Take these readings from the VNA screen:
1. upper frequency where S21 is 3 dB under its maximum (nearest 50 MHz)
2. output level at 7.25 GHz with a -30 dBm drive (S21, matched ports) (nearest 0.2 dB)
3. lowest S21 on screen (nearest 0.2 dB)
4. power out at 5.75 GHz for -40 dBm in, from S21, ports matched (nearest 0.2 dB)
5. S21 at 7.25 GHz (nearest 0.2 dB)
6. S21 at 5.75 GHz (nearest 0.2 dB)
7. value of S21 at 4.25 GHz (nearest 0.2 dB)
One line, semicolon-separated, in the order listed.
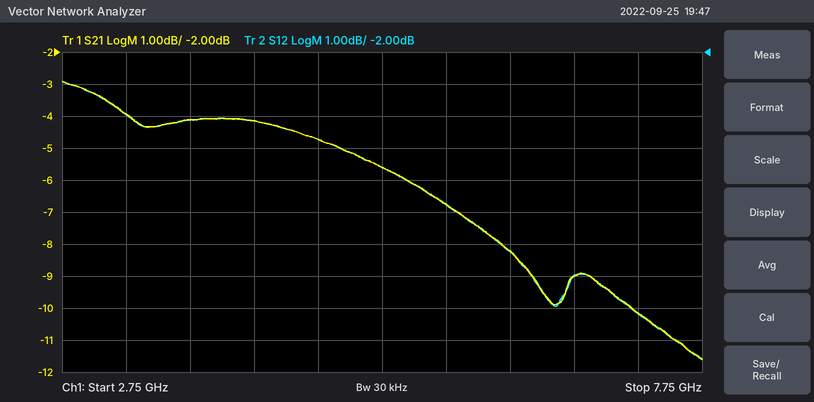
5.40 GHz; -40.2 dBm; -11.6 dB; -46.8 dBm; -10.2 dB; -6.8 dB; -4.2 dB
